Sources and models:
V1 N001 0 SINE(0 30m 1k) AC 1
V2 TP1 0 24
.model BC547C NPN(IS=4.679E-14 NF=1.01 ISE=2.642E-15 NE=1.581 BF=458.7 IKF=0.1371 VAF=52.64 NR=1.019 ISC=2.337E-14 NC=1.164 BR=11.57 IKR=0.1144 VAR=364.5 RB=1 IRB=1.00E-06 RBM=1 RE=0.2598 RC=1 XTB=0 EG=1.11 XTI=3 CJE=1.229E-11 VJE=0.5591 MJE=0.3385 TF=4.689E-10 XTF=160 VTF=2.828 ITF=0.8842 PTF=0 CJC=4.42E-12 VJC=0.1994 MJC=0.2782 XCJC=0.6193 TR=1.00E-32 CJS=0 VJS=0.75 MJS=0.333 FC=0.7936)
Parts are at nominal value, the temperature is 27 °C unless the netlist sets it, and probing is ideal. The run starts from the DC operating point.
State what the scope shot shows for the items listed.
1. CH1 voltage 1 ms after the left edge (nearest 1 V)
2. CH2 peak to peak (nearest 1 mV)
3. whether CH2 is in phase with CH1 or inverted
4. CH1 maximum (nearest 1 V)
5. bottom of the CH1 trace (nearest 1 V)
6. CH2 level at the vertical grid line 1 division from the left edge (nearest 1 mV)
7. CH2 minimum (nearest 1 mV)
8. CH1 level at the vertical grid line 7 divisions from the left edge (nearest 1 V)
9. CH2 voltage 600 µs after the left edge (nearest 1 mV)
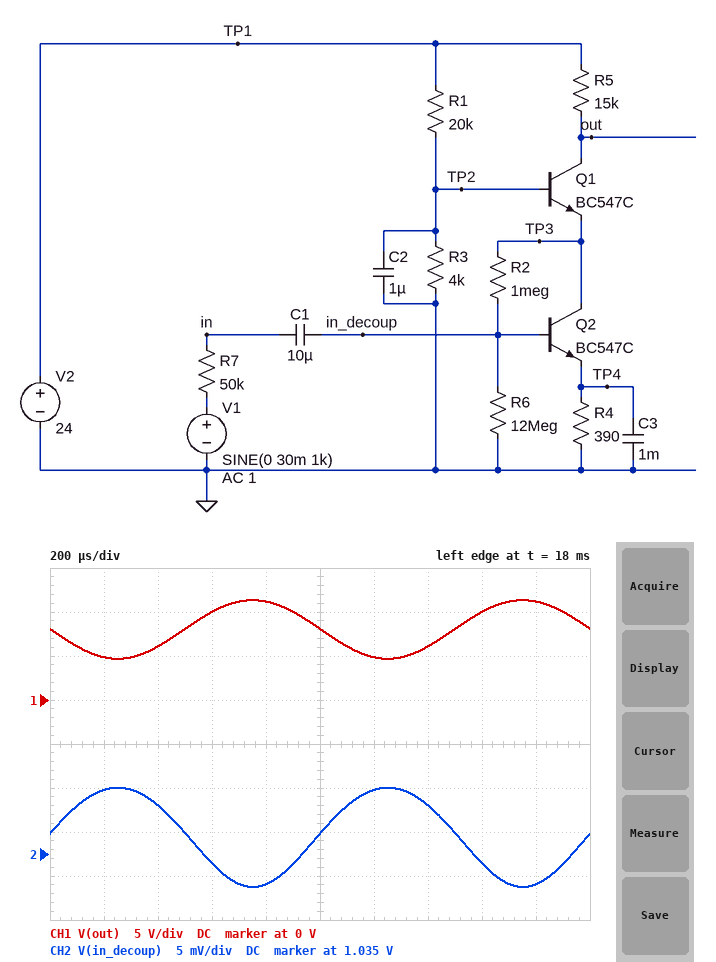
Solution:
8 V
11 mV
inverted
11 V
5 V
1.042 V
1.031 V
6 V
1.034 V
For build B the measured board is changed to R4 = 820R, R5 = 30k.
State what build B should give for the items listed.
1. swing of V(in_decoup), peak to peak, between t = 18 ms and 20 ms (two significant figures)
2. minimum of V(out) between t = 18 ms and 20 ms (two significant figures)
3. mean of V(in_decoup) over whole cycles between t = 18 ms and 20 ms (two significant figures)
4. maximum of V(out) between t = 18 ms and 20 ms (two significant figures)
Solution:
14 mV
3.0 V
1.3 V
6.5 V
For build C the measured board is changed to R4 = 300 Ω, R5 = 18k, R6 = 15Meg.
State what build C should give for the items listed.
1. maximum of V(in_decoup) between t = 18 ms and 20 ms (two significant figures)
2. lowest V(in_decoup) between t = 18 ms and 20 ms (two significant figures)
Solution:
960 mV
950 mV
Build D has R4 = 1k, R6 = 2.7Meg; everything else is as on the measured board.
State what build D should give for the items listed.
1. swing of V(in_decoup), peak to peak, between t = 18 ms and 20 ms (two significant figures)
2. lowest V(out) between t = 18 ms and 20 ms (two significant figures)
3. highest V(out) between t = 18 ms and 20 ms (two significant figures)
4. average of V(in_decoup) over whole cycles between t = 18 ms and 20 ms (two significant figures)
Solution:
15 mV
9.9 V
16 V
1.3 V
